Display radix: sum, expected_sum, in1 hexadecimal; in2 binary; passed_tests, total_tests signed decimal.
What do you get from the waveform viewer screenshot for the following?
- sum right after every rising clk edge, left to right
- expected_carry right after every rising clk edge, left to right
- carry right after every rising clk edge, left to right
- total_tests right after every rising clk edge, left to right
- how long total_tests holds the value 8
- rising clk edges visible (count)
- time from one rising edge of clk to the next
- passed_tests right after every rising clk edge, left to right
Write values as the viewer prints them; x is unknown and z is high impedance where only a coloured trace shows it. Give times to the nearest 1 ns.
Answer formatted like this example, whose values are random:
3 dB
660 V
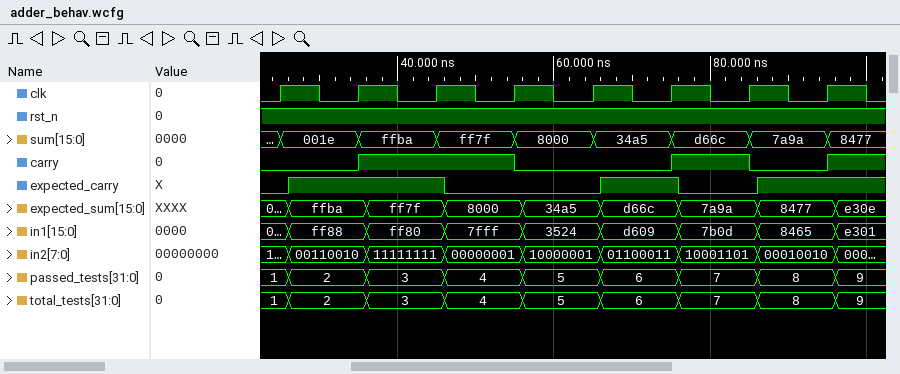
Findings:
001e, ffba, ff7f, 8000, 34a5, d66c, 7a9a, 8477
0 1 1 0 0 1 0 1
0 1 1 0 0 1 0 1
1, 2, 3, 4, 5, 6, 7, 8
10 ns
8
10 ns
1, 2, 3, 4, 5, 6, 7, 8
